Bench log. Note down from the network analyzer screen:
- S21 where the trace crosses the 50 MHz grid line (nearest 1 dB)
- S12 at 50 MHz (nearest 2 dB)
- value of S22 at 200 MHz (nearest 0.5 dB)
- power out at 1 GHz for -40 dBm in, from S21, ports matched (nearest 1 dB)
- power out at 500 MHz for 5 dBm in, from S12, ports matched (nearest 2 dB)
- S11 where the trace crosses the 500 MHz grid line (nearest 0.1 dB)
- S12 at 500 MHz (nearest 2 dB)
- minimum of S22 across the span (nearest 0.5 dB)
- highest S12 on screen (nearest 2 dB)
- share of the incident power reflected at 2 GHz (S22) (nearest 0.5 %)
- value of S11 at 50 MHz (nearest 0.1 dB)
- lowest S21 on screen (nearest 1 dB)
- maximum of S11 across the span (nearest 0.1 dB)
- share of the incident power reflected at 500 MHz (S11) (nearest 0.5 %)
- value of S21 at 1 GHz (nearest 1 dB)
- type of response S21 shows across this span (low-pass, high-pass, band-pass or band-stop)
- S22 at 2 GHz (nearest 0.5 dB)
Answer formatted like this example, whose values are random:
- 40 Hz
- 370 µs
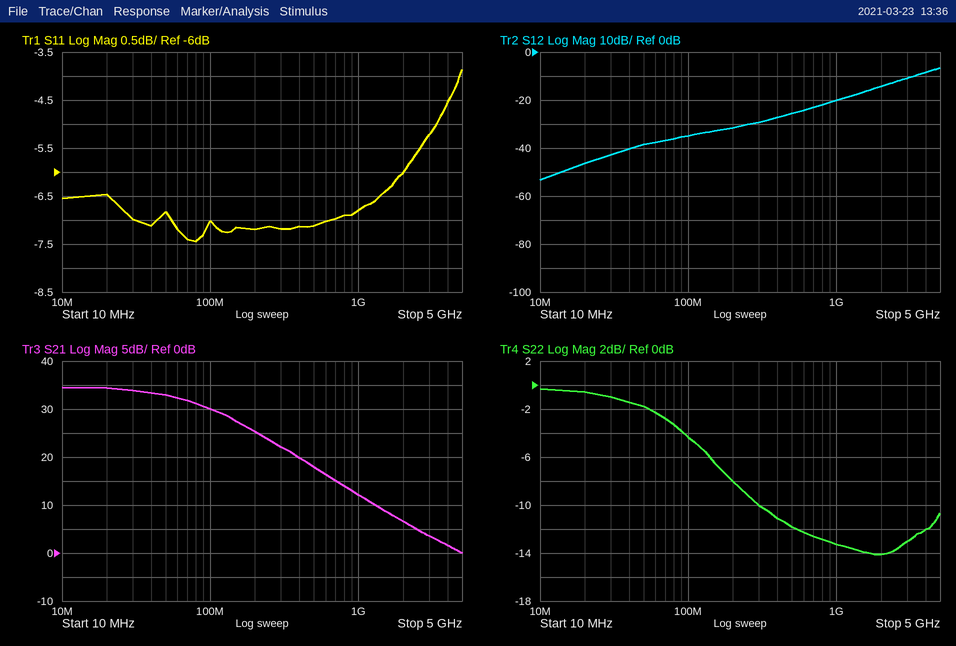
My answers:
- 33 dB
- -38 dB
- -8.0 dB
- -28 dBm
- -20 dBm
- -7.1 dB
- -26 dB
- -14.0 dB
- -6 dB
- 4.0 %
- -6.8 dB
- 0 dB
- -3.9 dB
- 19.5 %
- 12 dB
- low-pass
- -14.0 dB
